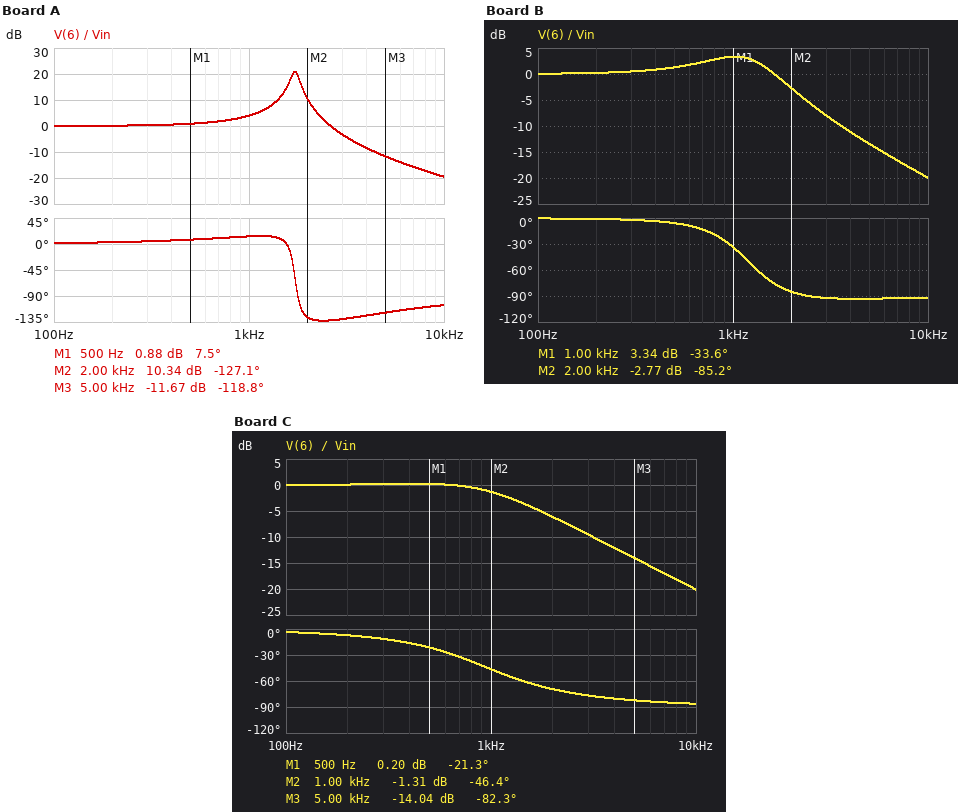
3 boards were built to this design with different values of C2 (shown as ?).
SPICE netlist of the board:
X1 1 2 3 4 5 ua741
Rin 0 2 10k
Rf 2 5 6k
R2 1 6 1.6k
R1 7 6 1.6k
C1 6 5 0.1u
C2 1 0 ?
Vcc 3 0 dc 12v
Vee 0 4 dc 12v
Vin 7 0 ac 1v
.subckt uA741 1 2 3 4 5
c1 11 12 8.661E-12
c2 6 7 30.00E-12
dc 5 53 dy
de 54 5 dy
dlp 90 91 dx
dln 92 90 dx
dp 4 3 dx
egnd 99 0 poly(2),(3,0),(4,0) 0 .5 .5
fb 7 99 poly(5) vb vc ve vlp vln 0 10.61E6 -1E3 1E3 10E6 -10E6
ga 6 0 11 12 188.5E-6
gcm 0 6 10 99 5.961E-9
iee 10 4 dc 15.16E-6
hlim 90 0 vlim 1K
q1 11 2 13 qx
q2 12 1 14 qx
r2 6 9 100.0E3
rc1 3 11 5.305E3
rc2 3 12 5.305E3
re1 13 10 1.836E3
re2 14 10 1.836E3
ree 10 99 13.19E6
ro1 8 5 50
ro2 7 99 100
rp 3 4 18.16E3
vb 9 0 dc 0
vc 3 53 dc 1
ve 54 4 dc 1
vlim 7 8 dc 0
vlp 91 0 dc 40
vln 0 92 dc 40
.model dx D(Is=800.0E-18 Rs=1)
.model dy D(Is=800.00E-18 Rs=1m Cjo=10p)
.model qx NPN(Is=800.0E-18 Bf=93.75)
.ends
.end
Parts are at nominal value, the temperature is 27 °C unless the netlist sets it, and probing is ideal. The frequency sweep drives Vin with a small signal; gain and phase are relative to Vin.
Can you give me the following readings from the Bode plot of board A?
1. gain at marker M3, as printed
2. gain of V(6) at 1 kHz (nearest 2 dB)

-11.67 dB
4 dB
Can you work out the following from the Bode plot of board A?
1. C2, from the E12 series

33 nF
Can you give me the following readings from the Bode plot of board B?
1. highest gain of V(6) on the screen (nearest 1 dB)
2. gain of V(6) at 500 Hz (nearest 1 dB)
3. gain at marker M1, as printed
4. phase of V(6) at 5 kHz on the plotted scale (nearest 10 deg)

3 dB
1 dB
3.34 dB
-90 deg
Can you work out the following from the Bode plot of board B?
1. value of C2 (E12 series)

68 nF
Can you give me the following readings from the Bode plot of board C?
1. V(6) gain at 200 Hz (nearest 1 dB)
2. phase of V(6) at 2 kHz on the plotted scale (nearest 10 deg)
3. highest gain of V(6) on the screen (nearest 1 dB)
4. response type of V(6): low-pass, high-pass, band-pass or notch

0 dB
-70 deg
0 dB
low-pass
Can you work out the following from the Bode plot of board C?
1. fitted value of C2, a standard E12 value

120 nF
